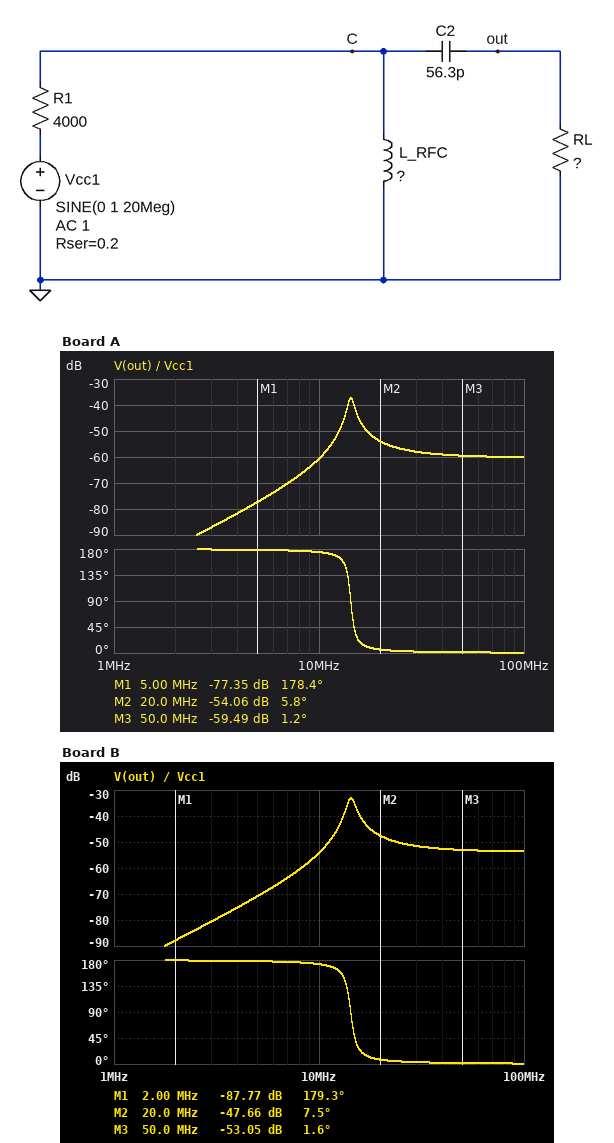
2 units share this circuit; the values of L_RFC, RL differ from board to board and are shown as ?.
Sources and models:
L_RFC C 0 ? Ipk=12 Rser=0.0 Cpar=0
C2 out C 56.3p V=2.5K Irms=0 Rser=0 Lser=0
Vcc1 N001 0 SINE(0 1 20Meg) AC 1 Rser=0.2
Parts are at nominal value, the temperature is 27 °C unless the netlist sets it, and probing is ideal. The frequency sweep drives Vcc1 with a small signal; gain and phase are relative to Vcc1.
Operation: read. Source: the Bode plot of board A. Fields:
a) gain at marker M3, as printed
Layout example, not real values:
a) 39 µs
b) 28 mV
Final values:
a) -59.49 dB
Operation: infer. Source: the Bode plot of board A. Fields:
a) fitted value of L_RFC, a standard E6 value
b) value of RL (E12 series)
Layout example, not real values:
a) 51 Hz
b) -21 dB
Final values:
a) 2.2 µH
b) 3.9 Ω
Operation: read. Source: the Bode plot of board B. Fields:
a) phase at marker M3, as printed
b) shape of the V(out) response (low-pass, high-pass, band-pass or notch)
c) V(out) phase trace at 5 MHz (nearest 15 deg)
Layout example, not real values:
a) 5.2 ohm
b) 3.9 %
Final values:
a) 1.6 deg
b) high-pass
c) 180 deg
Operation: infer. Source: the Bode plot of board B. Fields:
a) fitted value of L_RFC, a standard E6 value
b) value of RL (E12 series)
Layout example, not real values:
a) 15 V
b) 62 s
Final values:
a) 2.2 µH
b) 8.2 Ω
